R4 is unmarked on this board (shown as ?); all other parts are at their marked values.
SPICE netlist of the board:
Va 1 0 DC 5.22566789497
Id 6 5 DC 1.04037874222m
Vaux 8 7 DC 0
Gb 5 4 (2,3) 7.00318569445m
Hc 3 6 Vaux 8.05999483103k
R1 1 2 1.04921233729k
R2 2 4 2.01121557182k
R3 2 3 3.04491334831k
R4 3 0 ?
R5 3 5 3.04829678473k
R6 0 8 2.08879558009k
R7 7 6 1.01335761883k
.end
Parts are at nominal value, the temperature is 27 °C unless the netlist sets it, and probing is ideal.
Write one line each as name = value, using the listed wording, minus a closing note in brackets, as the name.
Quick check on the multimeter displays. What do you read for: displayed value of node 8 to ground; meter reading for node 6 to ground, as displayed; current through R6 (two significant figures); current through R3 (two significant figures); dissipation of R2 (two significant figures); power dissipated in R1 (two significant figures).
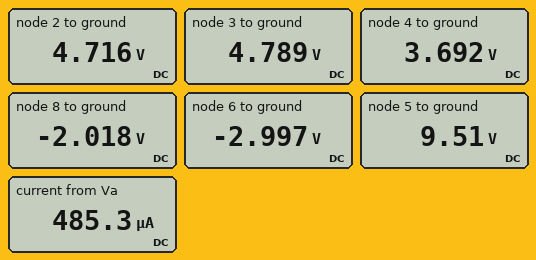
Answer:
displayed value of node 8 to ground = -2.018 V
meter reading for node 6 to ground, as displayed = -2.997 V
current through R6 = 970 µA
current through R3 = 24 µA
dissipation of R2 = 520 µW
power dissipated in R1 = 250 µW
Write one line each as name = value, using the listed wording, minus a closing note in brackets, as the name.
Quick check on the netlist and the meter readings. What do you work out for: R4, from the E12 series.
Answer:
R4, from the E12 series = 3.3 kΩ
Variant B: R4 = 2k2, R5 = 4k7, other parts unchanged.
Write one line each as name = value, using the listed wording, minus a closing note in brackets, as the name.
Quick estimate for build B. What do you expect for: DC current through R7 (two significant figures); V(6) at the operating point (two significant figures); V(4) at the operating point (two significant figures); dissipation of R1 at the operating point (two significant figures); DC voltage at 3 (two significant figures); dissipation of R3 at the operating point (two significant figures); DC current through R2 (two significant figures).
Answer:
DC current through R7 = 860 µA
V(6) at the operating point = -2.7 V
V(4) at the operating point = 1.8 V
dissipation of R1 at the operating point = 1.2 mW
DC voltage at 3 = 4.3 V
dissipation of R3 at the operating point = 8.5 µW
DC current through R2 = 1.1 mA
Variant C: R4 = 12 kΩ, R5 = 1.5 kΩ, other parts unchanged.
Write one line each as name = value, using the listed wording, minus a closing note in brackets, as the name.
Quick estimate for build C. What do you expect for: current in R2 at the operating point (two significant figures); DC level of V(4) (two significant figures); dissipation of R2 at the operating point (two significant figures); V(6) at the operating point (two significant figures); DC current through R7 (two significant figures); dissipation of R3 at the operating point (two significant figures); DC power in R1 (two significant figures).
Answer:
current in R2 at the operating point = 730 µA
DC level of V(4) = 7.4 V
dissipation of R2 at the operating point = 1.1 mW
V(6) at the operating point = -3.7 V
DC current through R7 = 1.2 mA
dissipation of R3 at the operating point = 3.5 µW
DC power in R1 = 500 µW
